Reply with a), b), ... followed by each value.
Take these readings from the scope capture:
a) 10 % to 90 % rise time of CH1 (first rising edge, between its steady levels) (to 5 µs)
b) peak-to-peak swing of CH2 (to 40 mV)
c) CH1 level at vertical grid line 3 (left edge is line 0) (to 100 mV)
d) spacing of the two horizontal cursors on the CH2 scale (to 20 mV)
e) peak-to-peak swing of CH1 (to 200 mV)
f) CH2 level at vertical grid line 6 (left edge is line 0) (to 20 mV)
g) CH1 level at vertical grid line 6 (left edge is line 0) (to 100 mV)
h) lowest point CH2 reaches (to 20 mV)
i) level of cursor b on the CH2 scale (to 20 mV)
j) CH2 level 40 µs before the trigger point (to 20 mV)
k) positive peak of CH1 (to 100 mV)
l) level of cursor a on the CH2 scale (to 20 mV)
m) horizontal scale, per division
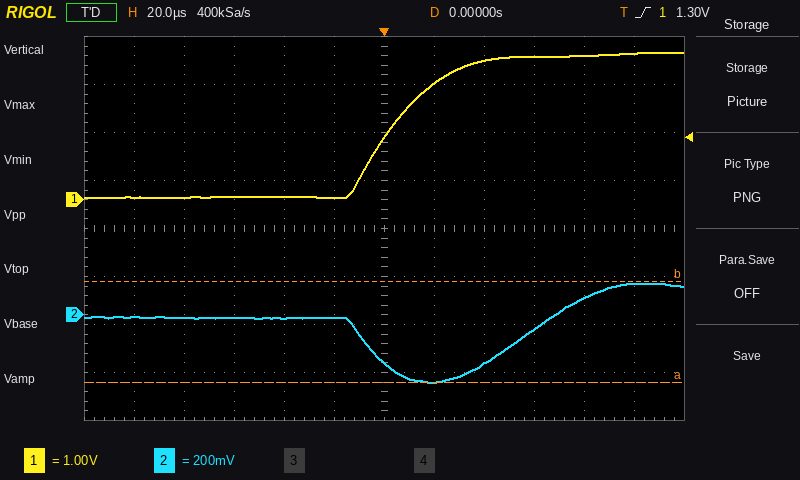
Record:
a) 40 µs
b) 400 mV
c) 100 mV
d) 420 mV
e) 3.0 V
f) -200 mV
g) 1.3 V
h) -280 mV
i) 140 mV
j) -20 mV
k) 3.1 V
l) -280 mV
m) 20 µs
